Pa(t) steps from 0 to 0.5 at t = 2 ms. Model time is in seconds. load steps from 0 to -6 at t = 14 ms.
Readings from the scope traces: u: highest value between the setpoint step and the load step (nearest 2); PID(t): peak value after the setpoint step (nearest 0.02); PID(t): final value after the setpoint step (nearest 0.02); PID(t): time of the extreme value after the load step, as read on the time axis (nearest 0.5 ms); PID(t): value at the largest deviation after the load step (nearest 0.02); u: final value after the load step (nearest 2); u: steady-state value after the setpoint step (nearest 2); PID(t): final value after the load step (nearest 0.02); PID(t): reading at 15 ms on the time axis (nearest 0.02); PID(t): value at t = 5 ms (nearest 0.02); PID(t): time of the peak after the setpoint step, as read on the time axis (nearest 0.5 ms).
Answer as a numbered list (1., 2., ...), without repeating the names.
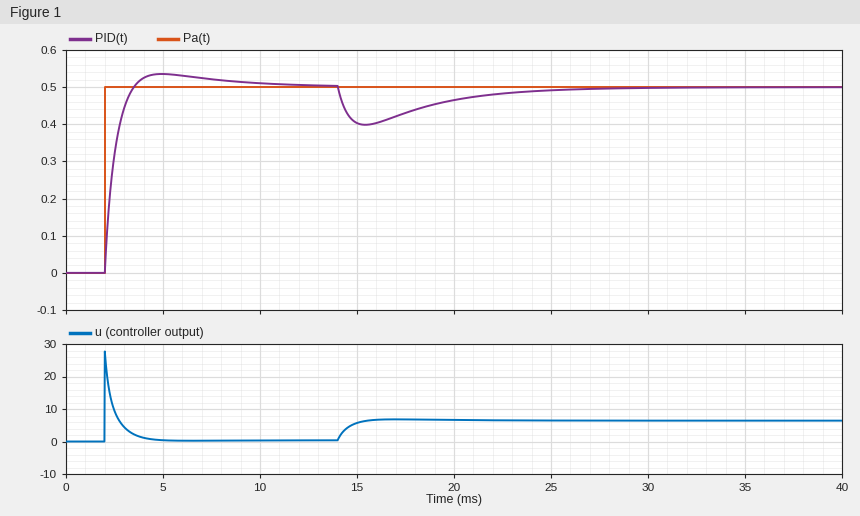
1. 28
2. 0.54
3. 0.50
4. 15.5 ms
5. 0.40
6. 6
7. 0
8. 0.50
9. 0.40
10. 0.54
11. 5.0 ms
